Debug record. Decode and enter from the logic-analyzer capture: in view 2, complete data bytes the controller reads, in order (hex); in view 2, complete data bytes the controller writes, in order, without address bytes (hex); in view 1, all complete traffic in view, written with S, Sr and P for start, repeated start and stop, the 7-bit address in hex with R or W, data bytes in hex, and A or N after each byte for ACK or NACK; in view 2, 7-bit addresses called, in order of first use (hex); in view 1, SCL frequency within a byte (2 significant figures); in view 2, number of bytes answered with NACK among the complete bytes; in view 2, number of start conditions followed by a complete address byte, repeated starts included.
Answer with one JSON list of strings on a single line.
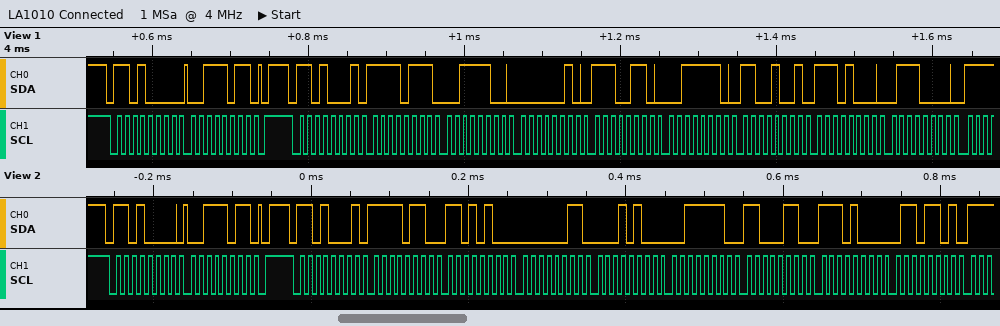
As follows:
["F6 D4 03 14 3E C6 E8 6D", "3B", "S 68W A 3B A P S 68R A F7 A 3C A 02 A E6 A 3E A C9 A E8 A 70 A", "0x68", "100 kHz", "0", "2"]
